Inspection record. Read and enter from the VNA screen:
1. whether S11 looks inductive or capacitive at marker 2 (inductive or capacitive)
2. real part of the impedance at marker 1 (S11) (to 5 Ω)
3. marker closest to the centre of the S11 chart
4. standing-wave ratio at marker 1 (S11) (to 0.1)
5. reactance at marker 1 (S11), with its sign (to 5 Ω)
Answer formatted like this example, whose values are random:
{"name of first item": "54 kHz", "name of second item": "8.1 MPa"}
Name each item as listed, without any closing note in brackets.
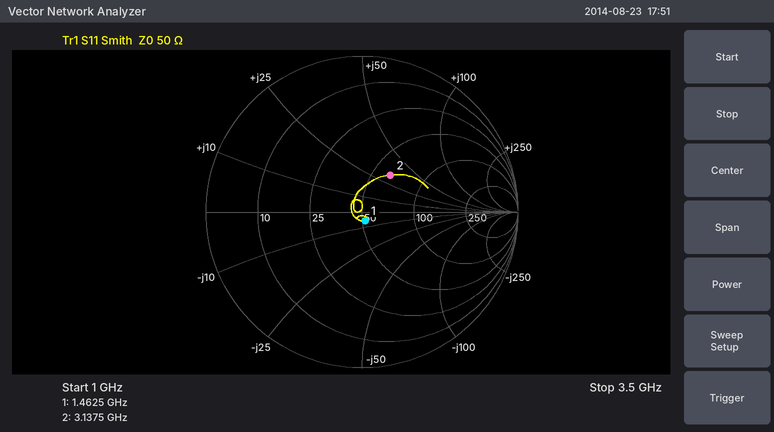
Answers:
{"whether S11 looks inductive or capacitive at marker 2": "inductive", "real part of the impedance at marker 1 (S11)": "50 Ω", "marker closest to the centre of the S11 chart": "marker 1", "standing-wave ratio at marker 1 (S11)": "1.1", "reactance at marker 1 (S11), with its sign": "-5 Ω"}
